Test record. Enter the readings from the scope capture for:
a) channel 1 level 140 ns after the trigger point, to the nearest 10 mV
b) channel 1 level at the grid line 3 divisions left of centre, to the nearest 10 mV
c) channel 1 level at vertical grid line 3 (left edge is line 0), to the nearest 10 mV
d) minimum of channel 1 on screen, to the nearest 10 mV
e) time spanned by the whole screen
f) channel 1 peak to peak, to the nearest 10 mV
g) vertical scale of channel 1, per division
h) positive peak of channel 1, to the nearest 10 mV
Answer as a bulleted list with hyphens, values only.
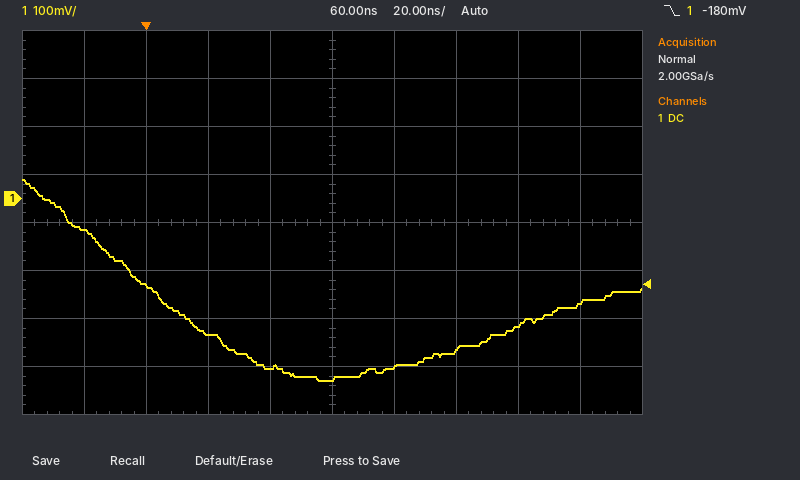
- -220 mV
- -180 mV
- -280 mV
- -380 mV
- 200 ns
- 420 mV
- 100 mV
- 40 mV
